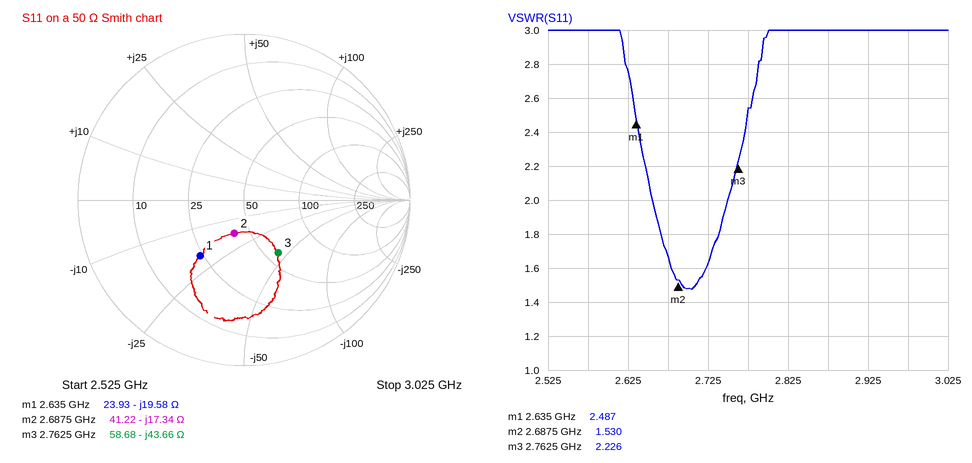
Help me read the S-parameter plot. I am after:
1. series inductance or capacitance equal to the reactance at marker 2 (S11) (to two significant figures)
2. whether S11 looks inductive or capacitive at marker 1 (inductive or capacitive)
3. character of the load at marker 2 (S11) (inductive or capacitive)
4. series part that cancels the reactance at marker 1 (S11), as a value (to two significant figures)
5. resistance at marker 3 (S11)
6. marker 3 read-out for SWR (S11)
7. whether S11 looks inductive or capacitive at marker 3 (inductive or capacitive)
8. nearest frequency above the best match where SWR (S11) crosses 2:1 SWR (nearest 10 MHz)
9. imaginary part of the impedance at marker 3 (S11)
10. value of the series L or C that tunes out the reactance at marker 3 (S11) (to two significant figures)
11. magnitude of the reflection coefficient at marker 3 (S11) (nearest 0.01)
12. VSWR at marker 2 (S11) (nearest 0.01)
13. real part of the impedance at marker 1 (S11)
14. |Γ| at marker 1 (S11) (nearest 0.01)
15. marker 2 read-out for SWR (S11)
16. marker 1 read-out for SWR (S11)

3.4 pF
capacitive
capacitive
1.2 nH
58.68 Ω
2.226
capacitive
2.75 GHz
-43.66 Ω
2.5 nH
0.38
1.53
23.93 Ω
0.43
1.530
2.487
